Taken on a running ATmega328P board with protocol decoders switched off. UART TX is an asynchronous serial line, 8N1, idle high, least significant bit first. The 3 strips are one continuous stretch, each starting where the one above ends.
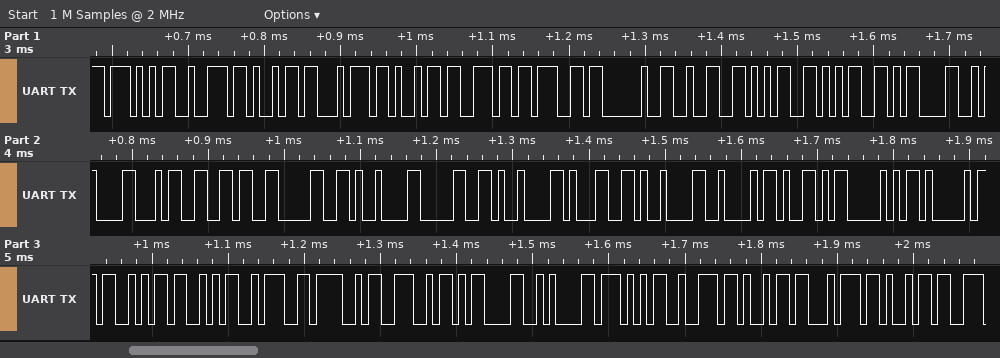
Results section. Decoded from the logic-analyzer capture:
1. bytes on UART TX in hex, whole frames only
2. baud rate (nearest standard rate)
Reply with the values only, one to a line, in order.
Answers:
57 72 69 74 69 6E 67 20 32 35 35 0D 0A 34 36 30 09 30 09 31 09 42 59 50 41 53 53 3A 4F 4E 0D 0A 57 72 69 74 69
115200 baud
